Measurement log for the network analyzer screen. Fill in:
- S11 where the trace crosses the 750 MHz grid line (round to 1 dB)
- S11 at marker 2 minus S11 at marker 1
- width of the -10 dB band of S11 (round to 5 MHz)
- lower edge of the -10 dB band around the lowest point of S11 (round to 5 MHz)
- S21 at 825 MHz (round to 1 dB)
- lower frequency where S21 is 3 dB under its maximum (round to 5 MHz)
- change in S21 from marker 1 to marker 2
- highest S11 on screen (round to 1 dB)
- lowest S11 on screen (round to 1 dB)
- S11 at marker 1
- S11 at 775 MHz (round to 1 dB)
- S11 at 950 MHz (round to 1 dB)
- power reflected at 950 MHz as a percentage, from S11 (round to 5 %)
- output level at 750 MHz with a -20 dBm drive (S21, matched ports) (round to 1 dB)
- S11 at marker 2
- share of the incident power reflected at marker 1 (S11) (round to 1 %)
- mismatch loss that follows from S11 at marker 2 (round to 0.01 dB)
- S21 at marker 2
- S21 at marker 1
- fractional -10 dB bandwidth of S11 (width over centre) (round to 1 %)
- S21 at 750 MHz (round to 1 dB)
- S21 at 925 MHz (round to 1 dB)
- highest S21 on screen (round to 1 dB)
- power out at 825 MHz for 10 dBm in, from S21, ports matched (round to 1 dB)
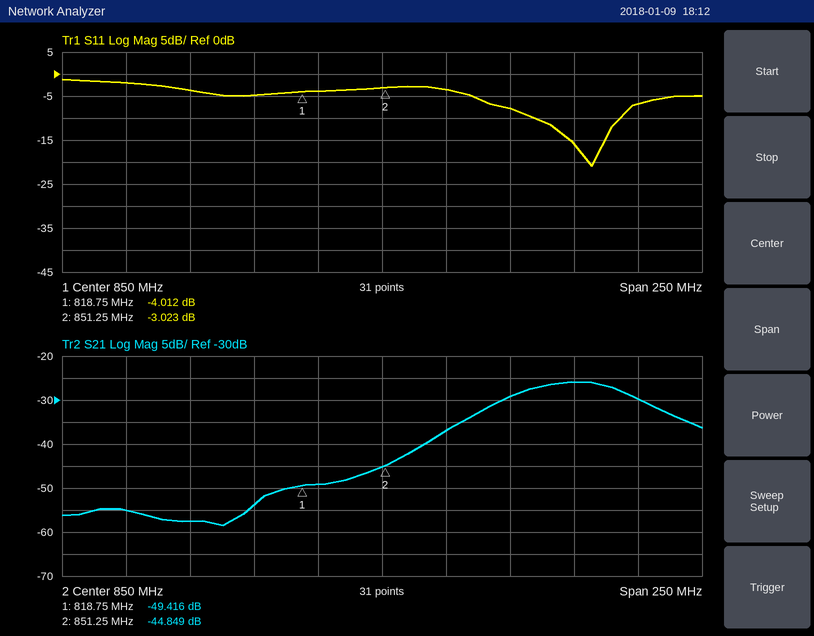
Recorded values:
-2 dB
0.989 dB
35 MHz
910 MHz
-49 dB
900 MHz
4.567 dB
-1 dB
-21 dB
-4.012 dB
-4 dB
-7 dB
20 %
-75 dBm
-3.023 dB
40 %
3.00 dB
-44.849 dB
-49.416 dB
4 %
-55 dB
-26 dB
-26 dB
-39 dBm
